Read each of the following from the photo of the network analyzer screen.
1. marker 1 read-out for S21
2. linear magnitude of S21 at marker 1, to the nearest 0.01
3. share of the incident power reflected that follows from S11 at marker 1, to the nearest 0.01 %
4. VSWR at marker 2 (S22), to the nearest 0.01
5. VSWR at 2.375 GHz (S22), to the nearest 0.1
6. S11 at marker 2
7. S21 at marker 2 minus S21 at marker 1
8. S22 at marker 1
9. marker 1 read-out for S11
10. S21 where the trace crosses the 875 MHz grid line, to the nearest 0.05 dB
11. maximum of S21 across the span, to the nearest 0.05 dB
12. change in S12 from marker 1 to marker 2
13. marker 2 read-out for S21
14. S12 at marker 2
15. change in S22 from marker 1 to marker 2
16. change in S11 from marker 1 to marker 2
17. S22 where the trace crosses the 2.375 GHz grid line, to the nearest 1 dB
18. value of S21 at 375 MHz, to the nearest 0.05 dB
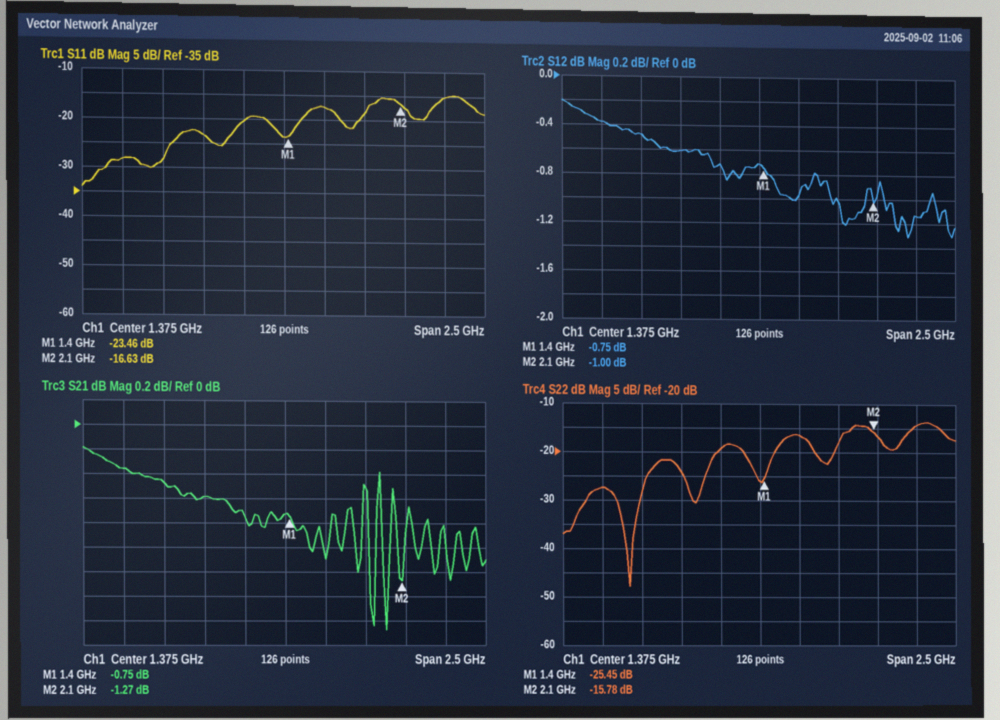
-0.75 dB
0.92
0.45 %
1.39
1.5
-16.63 dB
-0.52 dB
-25.45 dB
-23.46 dB
-0.60 dB
-0.20 dB
-0.25 dB
-1.27 dB
-1.00 dB
9.67 dB
6.83 dB
-14 dB
-0.35 dB
